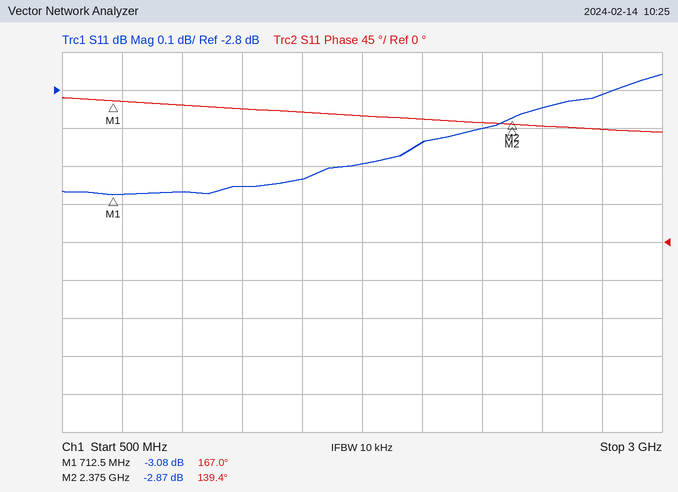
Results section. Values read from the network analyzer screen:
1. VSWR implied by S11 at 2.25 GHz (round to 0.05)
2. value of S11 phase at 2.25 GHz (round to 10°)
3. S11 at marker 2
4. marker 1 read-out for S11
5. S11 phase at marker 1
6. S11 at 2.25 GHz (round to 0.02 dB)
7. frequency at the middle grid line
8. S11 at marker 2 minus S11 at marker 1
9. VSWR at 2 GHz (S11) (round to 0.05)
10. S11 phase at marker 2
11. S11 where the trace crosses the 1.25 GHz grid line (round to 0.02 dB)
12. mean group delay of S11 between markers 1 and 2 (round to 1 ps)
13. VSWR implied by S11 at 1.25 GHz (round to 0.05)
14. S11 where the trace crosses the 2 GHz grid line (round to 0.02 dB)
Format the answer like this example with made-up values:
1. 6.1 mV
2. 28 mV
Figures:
1. 6.05
2. 140°
3. -2.87 dB
4. -3.08 dB
5. 167.0°
6. -2.90 dB
7. 1.75 GHz
8. 0.21 dB
9. 5.95
10. 139.4°
11. -3.06 dB
12. 46 ps
13. 5.75
14. -2.94 dB
